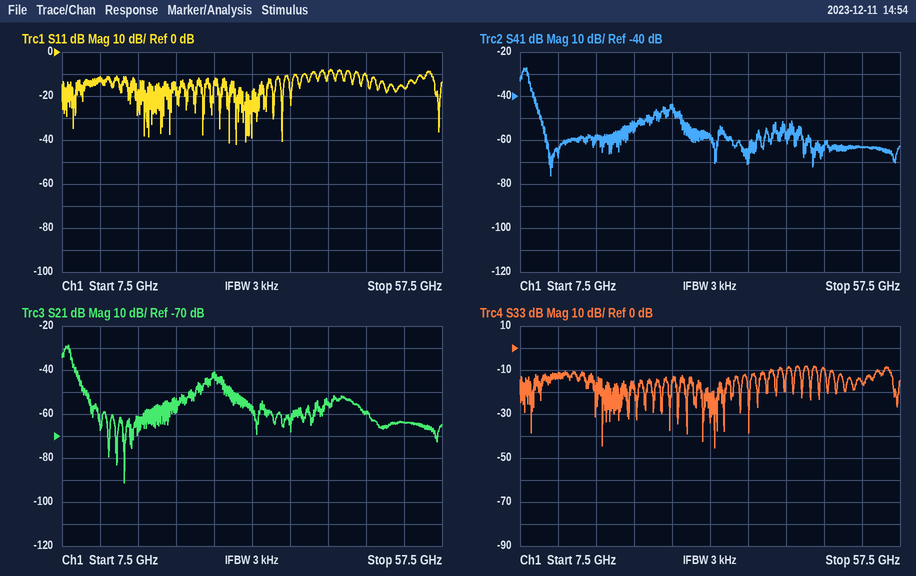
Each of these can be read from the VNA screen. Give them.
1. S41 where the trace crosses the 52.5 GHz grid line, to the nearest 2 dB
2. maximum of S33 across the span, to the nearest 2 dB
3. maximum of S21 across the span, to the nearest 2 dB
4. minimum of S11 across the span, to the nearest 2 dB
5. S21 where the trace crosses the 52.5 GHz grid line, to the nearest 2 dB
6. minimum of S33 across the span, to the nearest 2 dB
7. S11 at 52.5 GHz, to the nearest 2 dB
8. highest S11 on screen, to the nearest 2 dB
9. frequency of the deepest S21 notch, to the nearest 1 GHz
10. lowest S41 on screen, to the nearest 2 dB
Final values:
-64 dB
-8 dB
-28 dB
-42 dB
-64 dB
-46 dB
-16 dB
-8 dB
16 GHz
-76 dB
